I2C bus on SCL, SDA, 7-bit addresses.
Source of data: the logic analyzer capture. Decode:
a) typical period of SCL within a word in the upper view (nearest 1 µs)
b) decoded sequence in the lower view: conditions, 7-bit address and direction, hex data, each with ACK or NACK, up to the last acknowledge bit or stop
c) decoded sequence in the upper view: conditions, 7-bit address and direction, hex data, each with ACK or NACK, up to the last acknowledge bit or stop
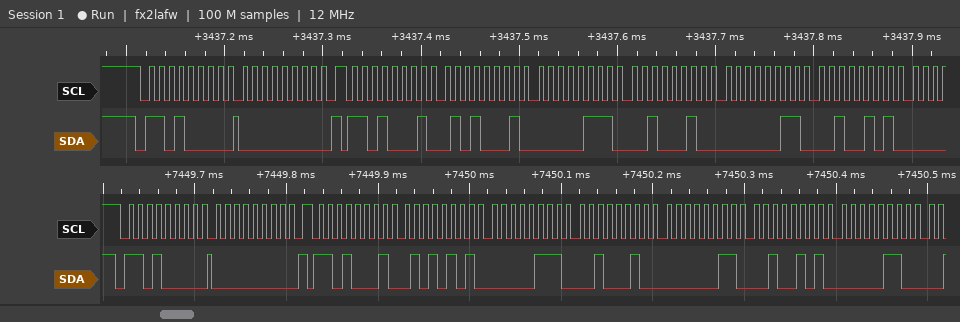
10 µs
start, address 68 write ACK, 00 ACK, repeated start, address 68 read ACK, 55 ACK, 07 ACK, 22 ACK, 03 ACK, 25 ACK, 06 ACK
start, address 68 write ACK, 00 ACK, repeated start, address 68 read ACK, 51 ACK, 07 ACK, 22 ACK, 03 ACK, 25 ACK
